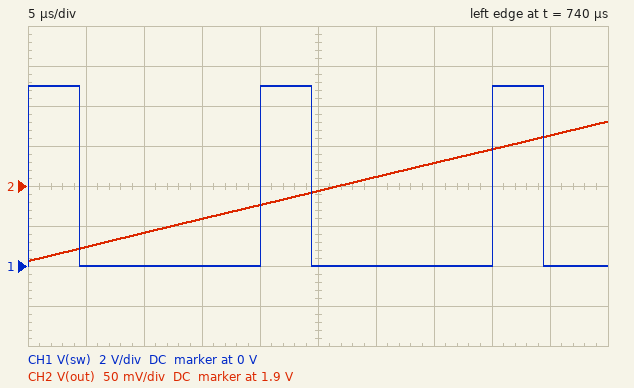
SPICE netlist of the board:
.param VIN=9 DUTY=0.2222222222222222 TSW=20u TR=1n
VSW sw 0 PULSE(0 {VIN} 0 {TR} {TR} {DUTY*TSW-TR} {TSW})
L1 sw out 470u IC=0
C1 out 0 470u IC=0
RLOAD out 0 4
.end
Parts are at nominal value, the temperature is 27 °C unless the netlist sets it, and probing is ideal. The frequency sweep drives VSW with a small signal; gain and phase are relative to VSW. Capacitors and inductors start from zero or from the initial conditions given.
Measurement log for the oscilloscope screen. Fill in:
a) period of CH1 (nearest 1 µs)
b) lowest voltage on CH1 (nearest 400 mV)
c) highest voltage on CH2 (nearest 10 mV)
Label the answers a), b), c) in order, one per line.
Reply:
a) 20 µs
b) 0 V
c) 1.98 V
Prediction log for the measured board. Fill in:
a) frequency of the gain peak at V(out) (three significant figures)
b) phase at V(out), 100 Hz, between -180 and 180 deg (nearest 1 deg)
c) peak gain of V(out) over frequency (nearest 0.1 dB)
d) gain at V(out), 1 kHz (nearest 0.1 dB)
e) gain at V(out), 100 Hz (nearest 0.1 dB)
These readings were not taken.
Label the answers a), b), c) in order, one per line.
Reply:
a) 333 Hz
b) -5 deg
c) 12.1 dB
d) -17.8 dB
e) 0.8 dB
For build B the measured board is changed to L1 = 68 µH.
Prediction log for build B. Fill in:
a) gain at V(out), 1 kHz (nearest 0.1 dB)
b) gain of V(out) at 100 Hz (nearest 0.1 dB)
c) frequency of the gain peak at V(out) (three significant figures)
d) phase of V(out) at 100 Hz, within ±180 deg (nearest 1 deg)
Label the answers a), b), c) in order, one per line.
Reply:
a) 11.0 dB
b) 0.1 dB
c) 888 Hz
d) -1 deg
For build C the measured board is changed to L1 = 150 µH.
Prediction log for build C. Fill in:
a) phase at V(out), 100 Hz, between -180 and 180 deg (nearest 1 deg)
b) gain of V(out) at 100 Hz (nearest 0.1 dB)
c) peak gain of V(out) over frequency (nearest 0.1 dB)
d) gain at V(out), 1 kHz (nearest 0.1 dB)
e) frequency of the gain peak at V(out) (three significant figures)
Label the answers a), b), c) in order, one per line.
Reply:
a) -1 deg
b) 0.2 dB
c) 17.0 dB
d) -5.1 dB
e) 596 Hz
